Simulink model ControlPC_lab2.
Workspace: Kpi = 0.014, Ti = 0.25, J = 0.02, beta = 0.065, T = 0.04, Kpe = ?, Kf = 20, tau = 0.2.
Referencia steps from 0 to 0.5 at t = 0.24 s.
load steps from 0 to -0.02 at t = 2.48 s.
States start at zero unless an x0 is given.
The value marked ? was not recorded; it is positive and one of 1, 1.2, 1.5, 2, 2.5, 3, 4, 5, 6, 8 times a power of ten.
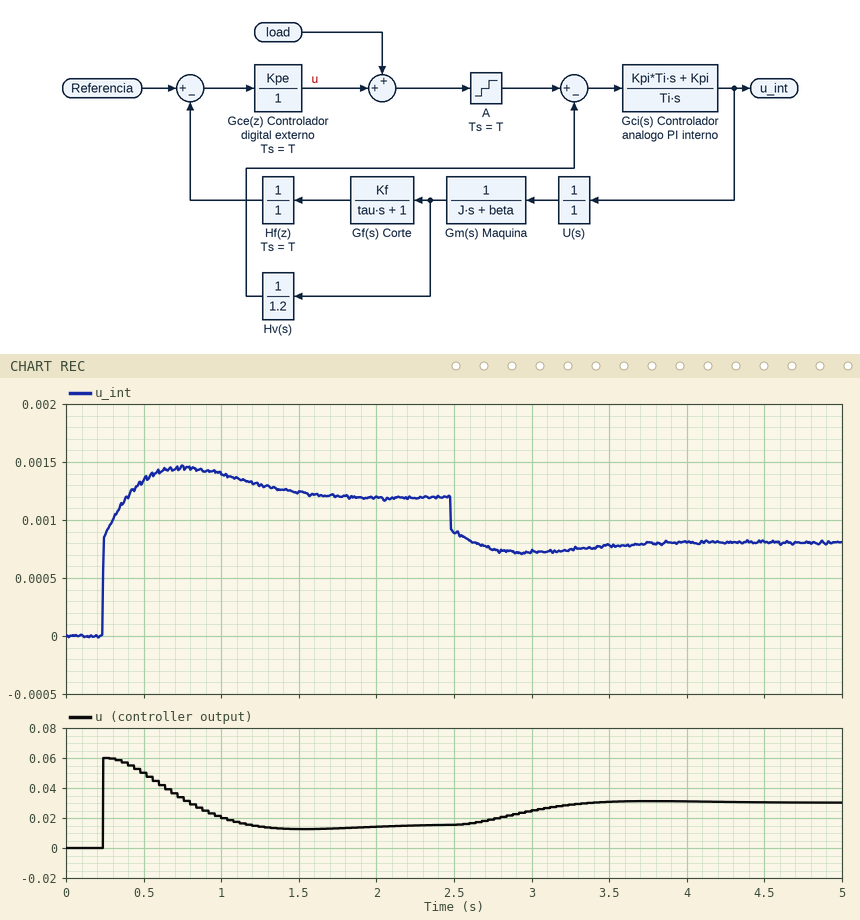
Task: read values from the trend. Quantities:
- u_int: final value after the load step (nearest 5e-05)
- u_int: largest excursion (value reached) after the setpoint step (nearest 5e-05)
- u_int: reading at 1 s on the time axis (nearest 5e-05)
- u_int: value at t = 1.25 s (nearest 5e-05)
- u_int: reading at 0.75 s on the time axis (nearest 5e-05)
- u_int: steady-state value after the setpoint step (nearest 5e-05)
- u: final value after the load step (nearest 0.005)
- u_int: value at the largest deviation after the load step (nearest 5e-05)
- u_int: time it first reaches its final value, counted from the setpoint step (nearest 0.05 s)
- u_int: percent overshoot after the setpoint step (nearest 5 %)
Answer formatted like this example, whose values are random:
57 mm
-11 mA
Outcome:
0.00080
0.00145
0.00140
0.00130
0.00145
0.00120
0.030
0.00070
0.15 s
20 %
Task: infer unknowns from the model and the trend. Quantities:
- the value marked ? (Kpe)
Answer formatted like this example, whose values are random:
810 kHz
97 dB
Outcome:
0.12
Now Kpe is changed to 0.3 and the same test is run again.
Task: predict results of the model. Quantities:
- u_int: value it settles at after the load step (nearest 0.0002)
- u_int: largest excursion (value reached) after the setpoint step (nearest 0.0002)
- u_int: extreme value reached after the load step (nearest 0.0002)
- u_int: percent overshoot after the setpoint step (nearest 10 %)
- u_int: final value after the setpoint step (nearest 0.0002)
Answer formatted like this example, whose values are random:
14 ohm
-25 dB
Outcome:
0.0012
0.0028
0.0010
100 %
0.0014
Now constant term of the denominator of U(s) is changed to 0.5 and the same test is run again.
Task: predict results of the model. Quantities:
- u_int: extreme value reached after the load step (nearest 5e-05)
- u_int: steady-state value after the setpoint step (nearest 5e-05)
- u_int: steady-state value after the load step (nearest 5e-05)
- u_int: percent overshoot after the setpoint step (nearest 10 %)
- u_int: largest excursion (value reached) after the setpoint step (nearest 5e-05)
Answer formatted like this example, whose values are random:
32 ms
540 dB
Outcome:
0.00025
0.00060
0.00040
80 %
0.00110
